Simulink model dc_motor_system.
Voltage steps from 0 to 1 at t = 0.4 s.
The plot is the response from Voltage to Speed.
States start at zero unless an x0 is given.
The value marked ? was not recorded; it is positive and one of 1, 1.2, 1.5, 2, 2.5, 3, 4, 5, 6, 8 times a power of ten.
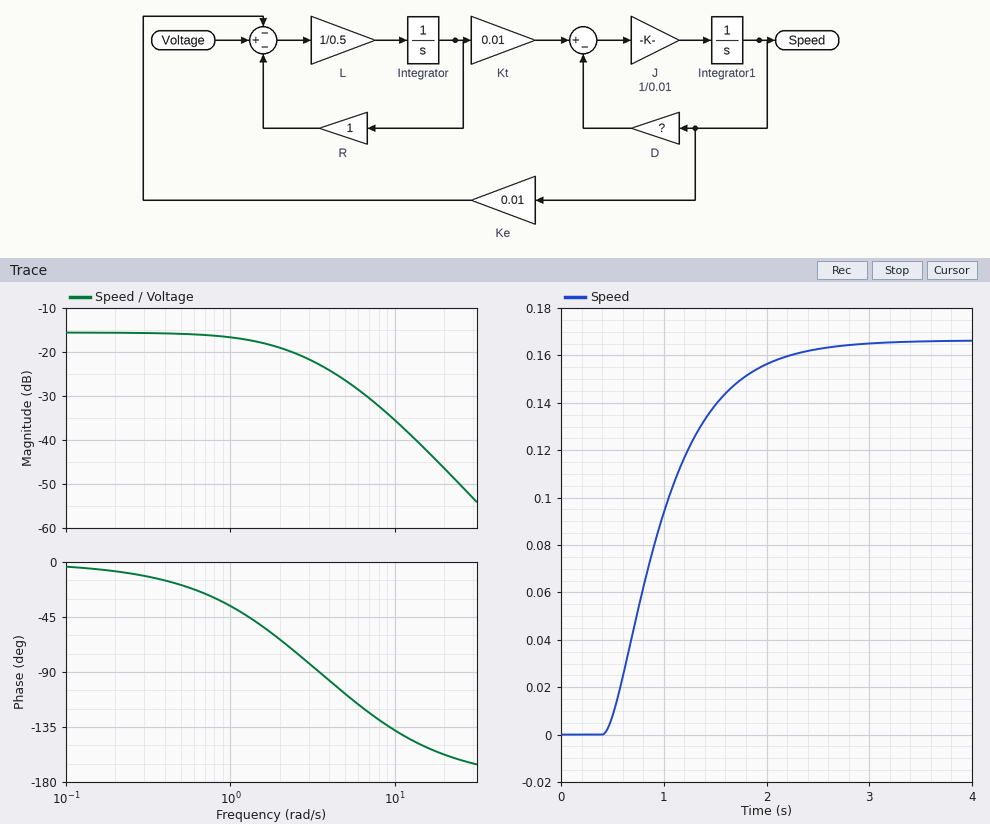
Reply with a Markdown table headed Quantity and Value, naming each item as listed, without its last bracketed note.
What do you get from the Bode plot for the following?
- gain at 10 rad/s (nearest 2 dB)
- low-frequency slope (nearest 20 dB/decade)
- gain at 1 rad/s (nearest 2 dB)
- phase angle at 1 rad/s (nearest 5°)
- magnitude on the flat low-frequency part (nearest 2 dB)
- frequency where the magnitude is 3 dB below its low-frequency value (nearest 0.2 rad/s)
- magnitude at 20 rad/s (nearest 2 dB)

| Quantity | Value |
|---|---|
| gain at 10 rad/s | -36 dB |
| low-frequency slope | 0 dB/decade |
| gain at 1 rad/s | -16 dB |
| phase angle at 1 rad/s | -35° |
| magnitude on the flat low-frequency part | -16 dB |
| frequency where the magnitude is 3 dB below its low-frequency value | 1.8 rad/s |
| magnitude at 20 rad/s | -46 dB |
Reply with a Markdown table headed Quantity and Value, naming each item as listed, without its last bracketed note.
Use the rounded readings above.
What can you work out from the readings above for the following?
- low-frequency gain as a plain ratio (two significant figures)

| Quantity | Value |
|---|---|
| low-frequency gain as a plain ratio | 0.16 |
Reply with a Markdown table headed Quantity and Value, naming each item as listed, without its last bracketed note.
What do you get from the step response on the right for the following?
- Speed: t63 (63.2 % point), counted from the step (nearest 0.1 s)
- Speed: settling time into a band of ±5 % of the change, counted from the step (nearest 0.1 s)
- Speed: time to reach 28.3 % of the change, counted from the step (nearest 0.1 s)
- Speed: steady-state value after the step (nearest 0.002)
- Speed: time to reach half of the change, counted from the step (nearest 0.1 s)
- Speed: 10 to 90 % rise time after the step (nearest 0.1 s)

| Quantity | Value |
|---|---|
| Speed: t63 (63.2 % point), counted from the step | 0.7 s |
| Speed: settling time into a band of ±5 % of the change, counted from the step | 1.7 s |
| Speed: time to reach 28.3 % of the change, counted from the step | 0.3 s |
| Speed: steady-state value after the step | 0.166 |
| Speed: time to reach half of the change, counted from the step | 0.5 s |
| Speed: 10 to 90 % rise time after the step | 1.2 s |
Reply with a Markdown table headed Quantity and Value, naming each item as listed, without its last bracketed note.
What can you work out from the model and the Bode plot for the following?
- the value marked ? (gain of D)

| Quantity | Value |
|---|---|
| the value marked ? | 0.06 |
